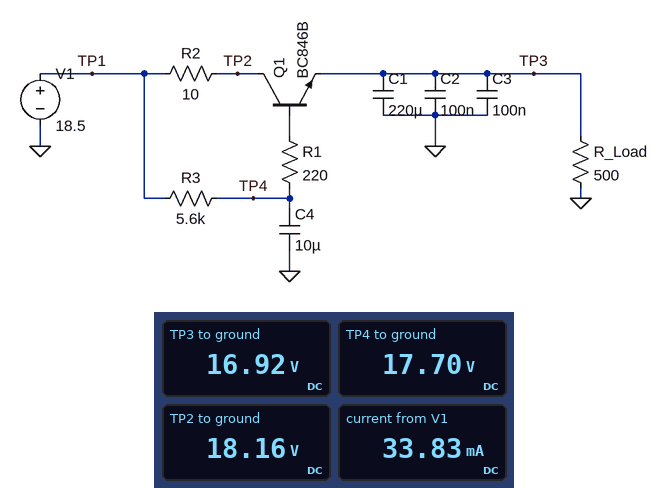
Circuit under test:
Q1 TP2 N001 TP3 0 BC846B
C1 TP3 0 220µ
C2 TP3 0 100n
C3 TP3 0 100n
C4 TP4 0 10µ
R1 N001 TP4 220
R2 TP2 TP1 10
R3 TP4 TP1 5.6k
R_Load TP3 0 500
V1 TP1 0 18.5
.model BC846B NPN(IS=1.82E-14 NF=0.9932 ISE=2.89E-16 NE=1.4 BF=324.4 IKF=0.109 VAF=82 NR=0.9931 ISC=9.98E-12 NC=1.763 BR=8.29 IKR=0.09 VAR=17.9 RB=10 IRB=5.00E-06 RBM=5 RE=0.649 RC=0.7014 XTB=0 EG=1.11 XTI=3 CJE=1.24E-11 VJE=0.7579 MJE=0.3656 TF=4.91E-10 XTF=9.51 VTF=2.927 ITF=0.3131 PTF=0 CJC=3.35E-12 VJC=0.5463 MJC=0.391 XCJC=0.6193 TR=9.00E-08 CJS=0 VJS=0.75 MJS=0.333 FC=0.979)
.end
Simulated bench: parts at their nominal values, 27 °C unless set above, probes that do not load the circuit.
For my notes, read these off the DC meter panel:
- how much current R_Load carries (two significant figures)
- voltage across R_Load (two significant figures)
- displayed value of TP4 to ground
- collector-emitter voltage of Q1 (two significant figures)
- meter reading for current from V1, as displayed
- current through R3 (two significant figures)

34 mA
17 V
17.70 V
1.2 V
33.83 mA
140 µA
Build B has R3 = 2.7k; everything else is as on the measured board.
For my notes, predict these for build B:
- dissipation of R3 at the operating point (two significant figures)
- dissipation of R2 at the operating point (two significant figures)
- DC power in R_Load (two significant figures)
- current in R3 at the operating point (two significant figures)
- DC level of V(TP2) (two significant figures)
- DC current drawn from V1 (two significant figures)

59 µW
12 mW
600 mW
150 µA
18 V
35 mA
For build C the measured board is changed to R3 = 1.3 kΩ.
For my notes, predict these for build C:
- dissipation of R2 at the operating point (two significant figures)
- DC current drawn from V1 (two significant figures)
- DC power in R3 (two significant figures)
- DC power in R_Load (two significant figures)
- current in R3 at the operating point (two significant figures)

12 mW
35 mA
29 µW
610 mW
150 µA
